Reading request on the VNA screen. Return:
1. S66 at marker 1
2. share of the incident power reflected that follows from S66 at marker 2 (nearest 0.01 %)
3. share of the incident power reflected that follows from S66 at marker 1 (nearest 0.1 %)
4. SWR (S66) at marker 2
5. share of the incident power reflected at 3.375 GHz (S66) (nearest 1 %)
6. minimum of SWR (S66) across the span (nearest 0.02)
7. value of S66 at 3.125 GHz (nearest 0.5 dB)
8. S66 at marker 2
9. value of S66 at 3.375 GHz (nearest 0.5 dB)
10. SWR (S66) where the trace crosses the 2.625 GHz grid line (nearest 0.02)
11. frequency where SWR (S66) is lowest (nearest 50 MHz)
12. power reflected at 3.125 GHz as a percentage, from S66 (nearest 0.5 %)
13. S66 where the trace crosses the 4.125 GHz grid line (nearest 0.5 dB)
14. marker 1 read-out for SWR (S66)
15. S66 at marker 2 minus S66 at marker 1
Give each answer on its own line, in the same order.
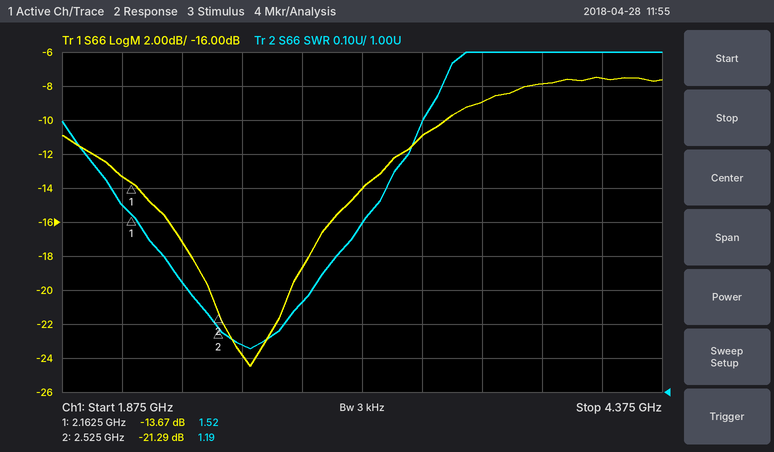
-13.67 dB
0.74 %
4.3 %
1.19
8 %
1.12
-14.0 dB
-21.29 dB
-11.0 dB
1.14
2.65 GHz
4.0 %
-7.5 dB
1.52
-7.62 dB
